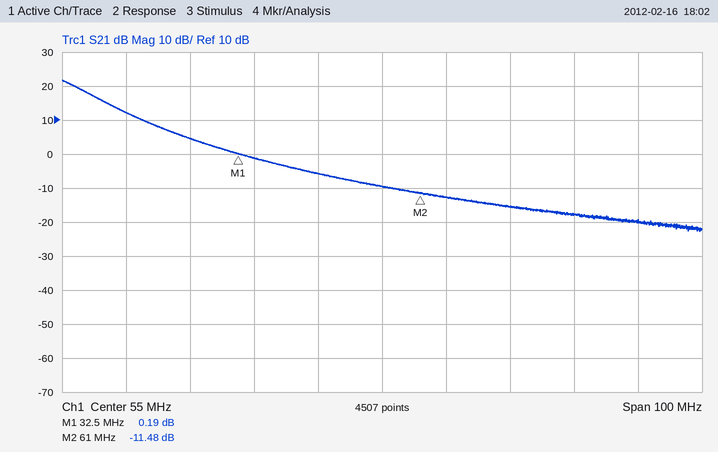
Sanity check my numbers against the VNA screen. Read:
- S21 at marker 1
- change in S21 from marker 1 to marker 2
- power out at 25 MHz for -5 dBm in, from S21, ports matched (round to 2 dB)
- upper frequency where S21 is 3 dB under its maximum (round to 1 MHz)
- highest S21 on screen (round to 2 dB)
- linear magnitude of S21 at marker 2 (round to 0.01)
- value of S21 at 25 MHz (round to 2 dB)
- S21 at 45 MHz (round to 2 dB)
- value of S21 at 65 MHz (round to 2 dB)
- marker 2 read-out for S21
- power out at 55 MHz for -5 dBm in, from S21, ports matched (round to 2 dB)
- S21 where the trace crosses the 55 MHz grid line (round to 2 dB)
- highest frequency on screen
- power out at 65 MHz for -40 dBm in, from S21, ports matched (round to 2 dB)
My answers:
0.19 dB
-11.67 dB
0 dBm
8 MHz
22 dB
0.27
4 dB
-6 dB
-12 dB
-11.48 dB
-14 dBm
-10 dB
105 MHz
-52 dBm
